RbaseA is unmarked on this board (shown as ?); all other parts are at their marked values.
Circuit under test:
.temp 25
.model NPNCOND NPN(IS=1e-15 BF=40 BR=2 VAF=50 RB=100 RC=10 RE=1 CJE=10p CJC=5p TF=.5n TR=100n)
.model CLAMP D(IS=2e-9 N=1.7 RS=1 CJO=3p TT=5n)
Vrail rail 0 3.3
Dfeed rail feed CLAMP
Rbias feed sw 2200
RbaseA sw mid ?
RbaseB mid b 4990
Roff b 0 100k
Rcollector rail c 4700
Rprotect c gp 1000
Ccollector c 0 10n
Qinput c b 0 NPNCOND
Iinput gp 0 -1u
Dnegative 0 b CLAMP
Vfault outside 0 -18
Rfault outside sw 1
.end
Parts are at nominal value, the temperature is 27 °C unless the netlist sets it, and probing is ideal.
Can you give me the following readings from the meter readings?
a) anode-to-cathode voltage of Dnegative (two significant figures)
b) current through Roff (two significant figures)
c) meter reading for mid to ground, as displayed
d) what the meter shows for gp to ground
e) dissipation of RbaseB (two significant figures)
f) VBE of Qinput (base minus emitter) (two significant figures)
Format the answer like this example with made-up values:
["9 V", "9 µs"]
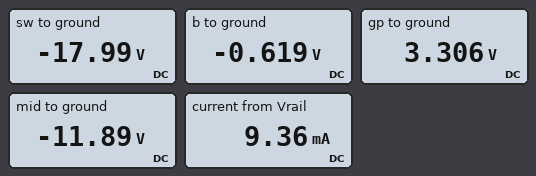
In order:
["620 mV", "6.2 µA", "-11.89 V", "3.306 V", "25 mW", "-620 mV"]
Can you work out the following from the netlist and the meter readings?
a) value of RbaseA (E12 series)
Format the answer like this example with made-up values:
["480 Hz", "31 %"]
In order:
["2.7 kΩ"]
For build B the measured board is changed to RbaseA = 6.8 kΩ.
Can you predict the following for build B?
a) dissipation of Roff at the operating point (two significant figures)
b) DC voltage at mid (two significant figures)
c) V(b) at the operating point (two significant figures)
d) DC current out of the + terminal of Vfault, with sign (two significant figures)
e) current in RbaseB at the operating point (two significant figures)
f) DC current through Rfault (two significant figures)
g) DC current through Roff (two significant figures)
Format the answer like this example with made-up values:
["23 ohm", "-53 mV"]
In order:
["3.6 µW", "-8.0 V", "-600 mV", "-11 mA", "1.5 mA", "11 mA", "6.0 µA"]
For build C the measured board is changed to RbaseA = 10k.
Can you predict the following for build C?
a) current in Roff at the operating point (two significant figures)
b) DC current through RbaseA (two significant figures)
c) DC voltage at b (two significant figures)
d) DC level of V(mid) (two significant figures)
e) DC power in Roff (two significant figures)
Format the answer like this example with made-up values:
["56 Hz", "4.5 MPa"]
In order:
["5.9 µA", "1.2 mA", "-590 mV", "-6.4 V", "3.5 µW"]
